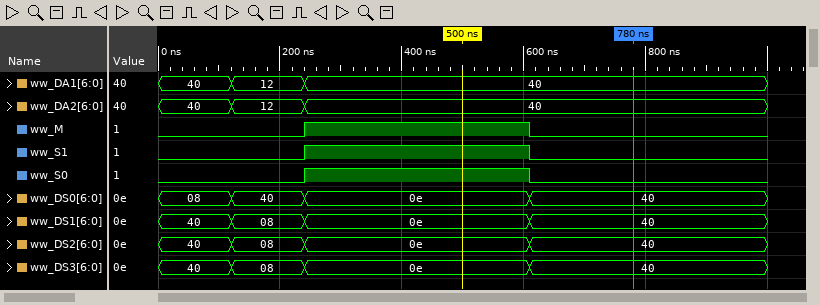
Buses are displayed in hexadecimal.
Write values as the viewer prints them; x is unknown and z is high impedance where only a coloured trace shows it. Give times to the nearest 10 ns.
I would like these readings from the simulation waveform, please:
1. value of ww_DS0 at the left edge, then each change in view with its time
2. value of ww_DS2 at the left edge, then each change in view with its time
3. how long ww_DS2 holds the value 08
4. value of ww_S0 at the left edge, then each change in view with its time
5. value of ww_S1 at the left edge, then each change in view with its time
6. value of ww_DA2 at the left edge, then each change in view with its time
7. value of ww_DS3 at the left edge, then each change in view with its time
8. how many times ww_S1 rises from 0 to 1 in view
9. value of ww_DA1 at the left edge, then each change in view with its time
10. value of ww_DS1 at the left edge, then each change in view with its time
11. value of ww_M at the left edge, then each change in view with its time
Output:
08, 40 at 120 ns, 0e at 240 ns, 40 at 610 ns
40, 08 at 120 ns, 0e at 240 ns, 40 at 610 ns
120 ns
0, 1 at 240 ns, 0 at 610 ns
0, 1 at 240 ns, 0 at 610 ns
40, 12 at 120 ns, 40 at 240 ns
40, 08 at 120 ns, 0e at 240 ns, 40 at 610 ns
1
40, 12 at 120 ns, 40 at 240 ns
40, 08 at 120 ns, 0e at 240 ns, 40 at 610 ns
0, 1 at 240 ns, 0 at 610 ns
